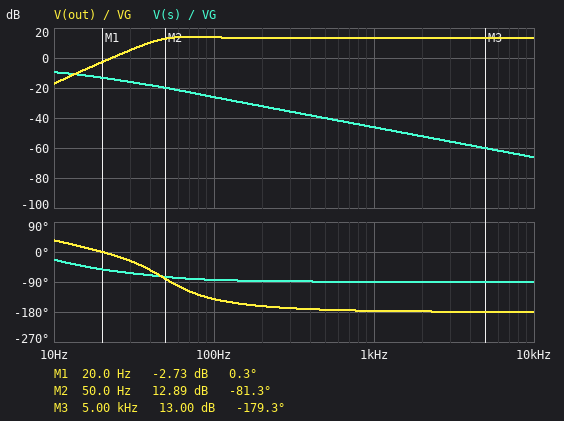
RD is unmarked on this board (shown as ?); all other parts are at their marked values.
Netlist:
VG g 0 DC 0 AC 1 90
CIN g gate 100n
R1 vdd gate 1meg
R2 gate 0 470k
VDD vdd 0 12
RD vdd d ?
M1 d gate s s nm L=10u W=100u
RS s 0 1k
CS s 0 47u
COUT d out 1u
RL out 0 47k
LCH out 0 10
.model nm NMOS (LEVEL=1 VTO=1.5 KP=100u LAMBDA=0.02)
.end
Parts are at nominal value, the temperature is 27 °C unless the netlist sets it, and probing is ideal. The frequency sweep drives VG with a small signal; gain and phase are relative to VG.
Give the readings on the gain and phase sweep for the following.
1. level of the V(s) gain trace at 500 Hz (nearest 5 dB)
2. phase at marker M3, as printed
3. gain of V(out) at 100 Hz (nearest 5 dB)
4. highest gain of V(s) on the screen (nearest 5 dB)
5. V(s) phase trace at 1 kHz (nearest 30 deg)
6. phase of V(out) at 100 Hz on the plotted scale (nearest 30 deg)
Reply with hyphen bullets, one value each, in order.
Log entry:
- -40 dB
- -179.3 deg
- 15 dB
- -10 dB
- -90 deg
- -150 deg
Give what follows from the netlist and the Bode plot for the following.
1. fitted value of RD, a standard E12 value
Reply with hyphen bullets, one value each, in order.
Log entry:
- 3.3 kΩ
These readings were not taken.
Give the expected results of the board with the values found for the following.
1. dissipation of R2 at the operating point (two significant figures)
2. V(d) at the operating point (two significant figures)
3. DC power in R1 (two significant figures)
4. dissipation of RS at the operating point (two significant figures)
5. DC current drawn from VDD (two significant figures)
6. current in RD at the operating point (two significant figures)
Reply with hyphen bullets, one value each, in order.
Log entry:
- 31 µW
- 8.7 V
- 67 µW
- 1.0 mW
- 1.0 mA
- 1.0 mA
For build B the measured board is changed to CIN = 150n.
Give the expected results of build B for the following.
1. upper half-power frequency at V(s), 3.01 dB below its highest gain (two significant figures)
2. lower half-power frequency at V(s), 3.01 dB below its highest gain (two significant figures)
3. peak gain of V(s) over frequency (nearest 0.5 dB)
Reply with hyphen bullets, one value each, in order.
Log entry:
- 14 Hz
- 2.0 Hz
- -7.5 dB
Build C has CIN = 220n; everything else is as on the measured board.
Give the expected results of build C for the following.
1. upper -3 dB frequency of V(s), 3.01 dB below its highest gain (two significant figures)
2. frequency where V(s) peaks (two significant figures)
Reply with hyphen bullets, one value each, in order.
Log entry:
- 12 Hz
- 4.3 Hz
